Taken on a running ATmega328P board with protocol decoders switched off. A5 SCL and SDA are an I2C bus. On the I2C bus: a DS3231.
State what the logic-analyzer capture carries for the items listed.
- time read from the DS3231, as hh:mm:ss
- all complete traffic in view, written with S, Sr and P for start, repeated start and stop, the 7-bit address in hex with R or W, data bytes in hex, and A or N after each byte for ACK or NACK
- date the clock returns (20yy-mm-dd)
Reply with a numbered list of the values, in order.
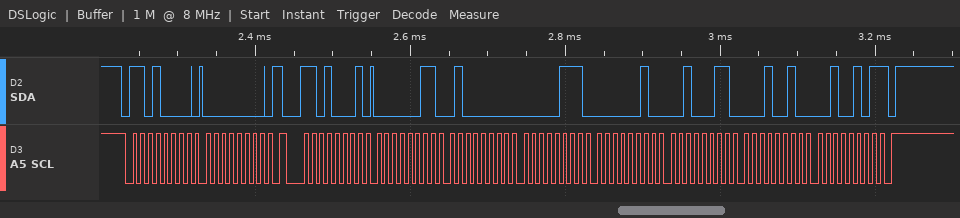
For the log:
1. 07:40:03
2. S 68W A 00 A Sr 68R A 03 A 40 A 07 A 02 A 23 A 12 A 25 N P
3. 2025-12-23
